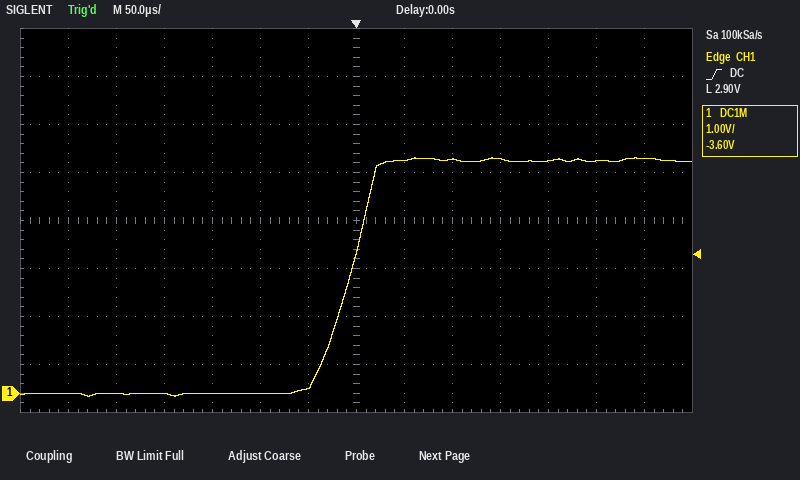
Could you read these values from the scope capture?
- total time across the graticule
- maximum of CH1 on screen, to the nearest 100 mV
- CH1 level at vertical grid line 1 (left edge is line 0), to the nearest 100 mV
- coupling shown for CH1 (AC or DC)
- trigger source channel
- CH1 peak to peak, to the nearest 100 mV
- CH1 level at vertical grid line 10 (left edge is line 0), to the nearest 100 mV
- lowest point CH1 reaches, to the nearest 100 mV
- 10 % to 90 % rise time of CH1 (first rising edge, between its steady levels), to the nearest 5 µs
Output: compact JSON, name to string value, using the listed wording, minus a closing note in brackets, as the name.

{"total time across the graticule": "700 µs", "maximum of CH1 on screen, to the nearest 100 mV": "4.9 V", "CH1 level at vertical grid line 1 (left edge is line 0), to the nearest 100 mV": "0.0 V", "coupling shown for CH1": "DC", "trigger source channel": "CH1", "CH1 peak to peak, to the nearest 100 mV": "5.0 V", "CH1 level at vertical grid line 10 (left edge is line 0), to the nearest 100 mV": "4.9 V", "lowest point CH1 reaches, to the nearest 100 mV": "-100 mV", "10 % to 90 % rise time of CH1 (first rising edge, between its steady levels), to the nearest 5 µs": "55 µs"}
